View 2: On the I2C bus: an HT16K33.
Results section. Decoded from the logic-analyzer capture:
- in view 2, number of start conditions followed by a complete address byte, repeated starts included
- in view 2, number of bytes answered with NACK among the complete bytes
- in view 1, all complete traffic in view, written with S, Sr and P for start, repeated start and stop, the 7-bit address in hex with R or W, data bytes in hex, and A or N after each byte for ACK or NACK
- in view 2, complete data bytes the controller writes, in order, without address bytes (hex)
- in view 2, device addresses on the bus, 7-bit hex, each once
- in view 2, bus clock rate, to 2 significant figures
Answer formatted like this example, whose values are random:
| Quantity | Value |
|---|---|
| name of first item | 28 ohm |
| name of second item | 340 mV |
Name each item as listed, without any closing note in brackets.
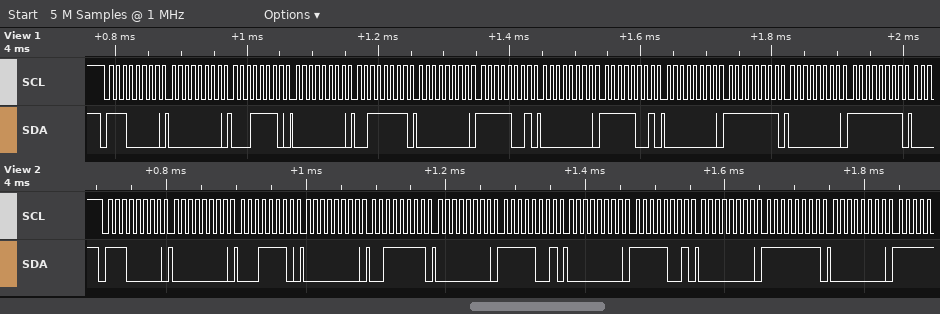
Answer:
| Quantity | Value |
|---|---|
| in view 2, number of start conditions followed by a complete address byte, repeated starts included | 1 |
| in view 2, number of bytes answered with NACK among the complete bytes | 0 |
| in view 1, all complete traffic in view, written with S, Sr and P for start, repeated start and stop, the 7-bit address in hex with R or W, data bytes in hex, and A or N after each byte for ACK or NACK | S 70W A 00 A 1E A 00 A 3F A 00 A F9 A 00 A F9 A 00 A FF A 00 A FF A |
| in view 2, complete data bytes the controller writes, in order, without address bytes | 00 1E 00 3F 00 F9 00 F9 00 FF 00 |
| in view 2, device addresses on the bus, 7-bit hex, each once | 0x70 |
| in view 2, bus clock rate, to 2 significant figures | 100 kHz |
